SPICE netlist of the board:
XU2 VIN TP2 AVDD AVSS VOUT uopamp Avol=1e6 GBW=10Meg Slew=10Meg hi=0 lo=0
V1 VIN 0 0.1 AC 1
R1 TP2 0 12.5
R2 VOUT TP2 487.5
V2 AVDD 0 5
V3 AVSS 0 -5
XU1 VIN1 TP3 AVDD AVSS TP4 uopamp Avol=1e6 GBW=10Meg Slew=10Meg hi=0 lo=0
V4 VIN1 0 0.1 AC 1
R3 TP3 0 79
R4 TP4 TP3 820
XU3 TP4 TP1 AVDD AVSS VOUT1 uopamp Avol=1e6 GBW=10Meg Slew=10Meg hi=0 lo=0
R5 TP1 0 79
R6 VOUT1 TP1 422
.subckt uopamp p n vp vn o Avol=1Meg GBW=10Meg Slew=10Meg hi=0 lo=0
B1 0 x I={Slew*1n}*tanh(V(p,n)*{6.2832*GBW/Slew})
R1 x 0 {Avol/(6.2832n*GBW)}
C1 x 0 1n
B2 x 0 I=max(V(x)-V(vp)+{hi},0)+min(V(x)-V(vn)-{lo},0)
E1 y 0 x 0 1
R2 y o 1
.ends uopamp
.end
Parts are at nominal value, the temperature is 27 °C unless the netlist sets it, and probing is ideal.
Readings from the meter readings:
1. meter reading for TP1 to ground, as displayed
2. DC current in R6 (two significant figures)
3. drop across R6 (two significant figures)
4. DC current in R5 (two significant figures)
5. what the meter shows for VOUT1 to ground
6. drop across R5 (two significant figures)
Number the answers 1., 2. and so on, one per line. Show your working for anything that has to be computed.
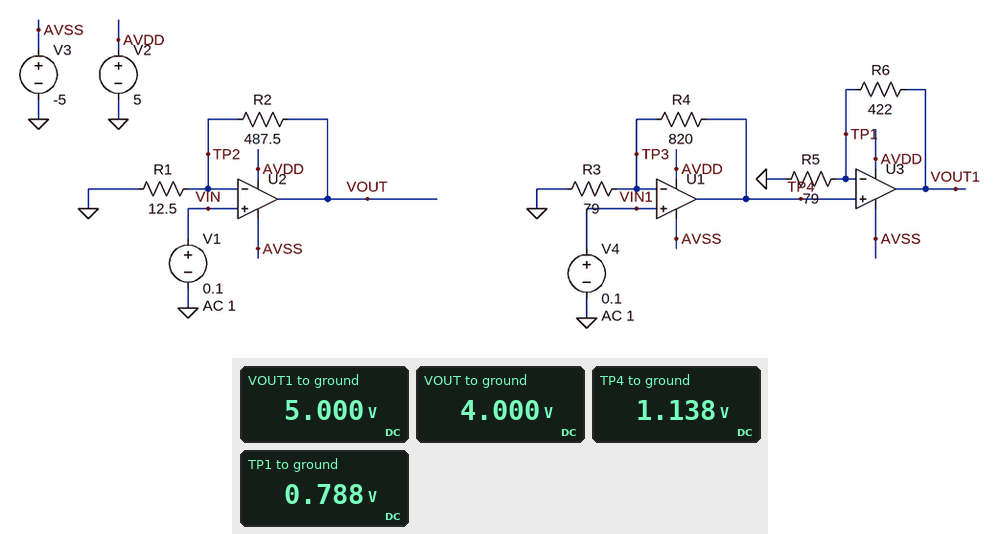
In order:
1. 0.788 V
2. (5 V - 788 mV) / 422 Ω = 10 mA
3. 5 V - 788 mV = 4.2 V
4. (788 mV) / 79 Ω = 10 mA
5. 5.000 V
6. 788 mV = 790 mV
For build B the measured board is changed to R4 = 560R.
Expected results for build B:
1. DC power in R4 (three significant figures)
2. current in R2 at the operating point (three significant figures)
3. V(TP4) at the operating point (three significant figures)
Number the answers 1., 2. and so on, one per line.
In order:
1. 897 µW
2. 8.00 mA
3. 809 mV
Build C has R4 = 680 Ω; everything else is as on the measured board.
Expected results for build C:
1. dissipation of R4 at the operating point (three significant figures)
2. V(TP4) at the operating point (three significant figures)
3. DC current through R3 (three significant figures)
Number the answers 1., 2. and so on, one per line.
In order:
1. 1.09 mW
2. 961 mV
3. 1.27 mA
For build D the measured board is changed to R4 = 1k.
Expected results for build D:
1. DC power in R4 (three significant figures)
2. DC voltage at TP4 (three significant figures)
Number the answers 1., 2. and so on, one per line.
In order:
1. 1.60 mW
2. 1.37 V
